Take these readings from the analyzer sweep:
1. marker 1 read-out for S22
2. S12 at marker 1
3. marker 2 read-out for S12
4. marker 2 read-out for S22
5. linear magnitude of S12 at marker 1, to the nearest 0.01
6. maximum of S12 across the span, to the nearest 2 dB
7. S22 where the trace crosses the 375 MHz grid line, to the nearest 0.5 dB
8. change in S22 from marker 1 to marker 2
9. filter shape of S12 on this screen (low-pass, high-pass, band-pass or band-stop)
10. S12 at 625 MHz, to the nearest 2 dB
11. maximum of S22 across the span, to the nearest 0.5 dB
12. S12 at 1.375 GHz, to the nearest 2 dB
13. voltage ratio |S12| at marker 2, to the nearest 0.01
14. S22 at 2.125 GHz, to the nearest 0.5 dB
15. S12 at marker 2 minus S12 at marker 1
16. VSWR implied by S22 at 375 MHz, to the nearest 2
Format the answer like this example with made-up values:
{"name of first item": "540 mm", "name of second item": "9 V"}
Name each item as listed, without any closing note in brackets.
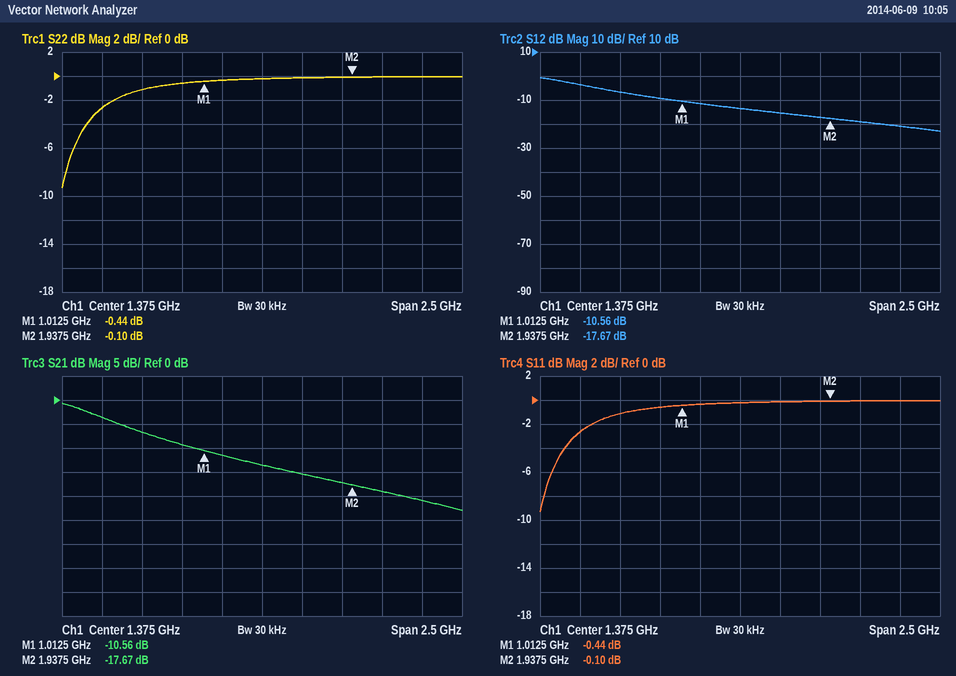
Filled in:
{"marker 1 read-out for S22": "-0.44 dB", "S12 at marker 1": "-10.56 dB", "marker 2 read-out for S12": "-17.67 dB", "marker 2 read-out for S22": "-0.10 dB", "linear magnitude of S12 at marker 1, to the nearest 0.01": "0.30", "maximum of S12 across the span, to the nearest 2 dB": "0 dB", "S22 where the trace crosses the 375 MHz grid line, to the nearest 0.5 dB": "-2.5 dB", "change in S22 from marker 1 to marker 2": "0.34 dB", "filter shape of S12 on this screen": "low-pass", "S12 at 625 MHz, to the nearest 2 dB": "-6 dB", "maximum of S22 across the span, to the nearest 0.5 dB": "0.0 dB", "S12 at 1.375 GHz, to the nearest 2 dB": "-14 dB", "voltage ratio |S12| at marker 2, to the nearest 0.01": "0.13", "S22 at 2.125 GHz, to the nearest 0.5 dB": "0.0 dB", "S12 at marker 2 minus S12 at marker 1": "-7.11 dB", "VSWR implied by S22 at 375 MHz, to the nearest 2": "6"}
